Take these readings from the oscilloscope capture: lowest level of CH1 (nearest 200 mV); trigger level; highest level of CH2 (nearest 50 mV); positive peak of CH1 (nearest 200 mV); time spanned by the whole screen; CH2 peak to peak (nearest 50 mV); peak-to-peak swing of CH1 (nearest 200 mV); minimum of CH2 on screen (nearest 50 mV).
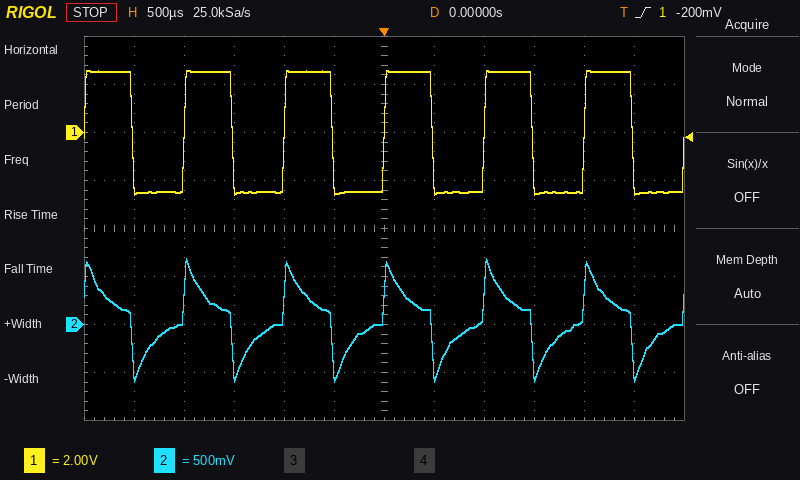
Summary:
-2.6 V
-200 mV
700 mV
2.6 V
6 ms
1.30 V
5.2 V
-600 mV
